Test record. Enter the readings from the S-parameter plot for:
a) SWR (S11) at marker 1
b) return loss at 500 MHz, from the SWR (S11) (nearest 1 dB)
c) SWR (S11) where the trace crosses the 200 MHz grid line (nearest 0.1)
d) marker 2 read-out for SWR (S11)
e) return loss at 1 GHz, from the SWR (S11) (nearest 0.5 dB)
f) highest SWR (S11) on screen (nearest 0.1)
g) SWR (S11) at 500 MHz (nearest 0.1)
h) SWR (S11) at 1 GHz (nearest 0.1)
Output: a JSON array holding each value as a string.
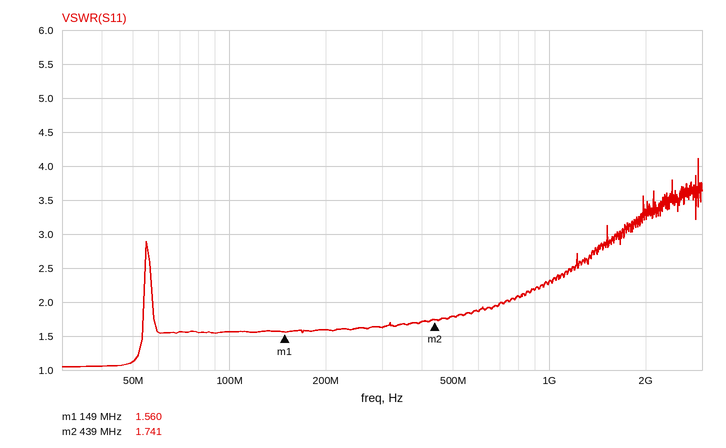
["1.560", "11 dB", "1.6", "1.741", "8.0 dB", "4.1", "1.8", "2.3"]
